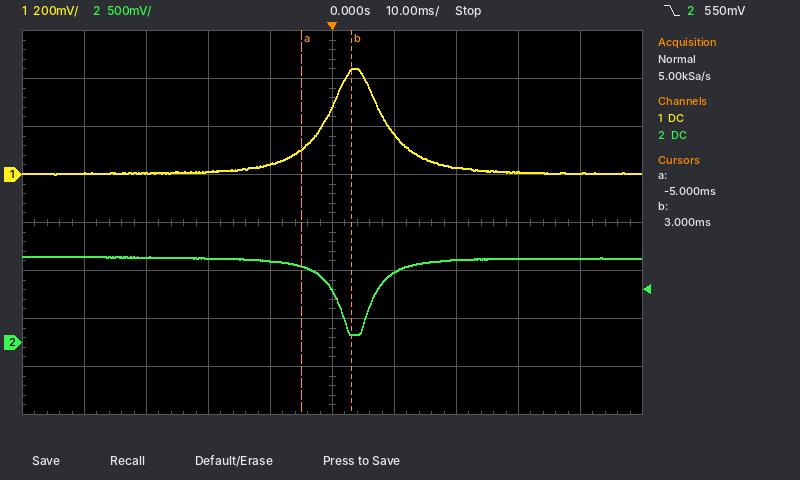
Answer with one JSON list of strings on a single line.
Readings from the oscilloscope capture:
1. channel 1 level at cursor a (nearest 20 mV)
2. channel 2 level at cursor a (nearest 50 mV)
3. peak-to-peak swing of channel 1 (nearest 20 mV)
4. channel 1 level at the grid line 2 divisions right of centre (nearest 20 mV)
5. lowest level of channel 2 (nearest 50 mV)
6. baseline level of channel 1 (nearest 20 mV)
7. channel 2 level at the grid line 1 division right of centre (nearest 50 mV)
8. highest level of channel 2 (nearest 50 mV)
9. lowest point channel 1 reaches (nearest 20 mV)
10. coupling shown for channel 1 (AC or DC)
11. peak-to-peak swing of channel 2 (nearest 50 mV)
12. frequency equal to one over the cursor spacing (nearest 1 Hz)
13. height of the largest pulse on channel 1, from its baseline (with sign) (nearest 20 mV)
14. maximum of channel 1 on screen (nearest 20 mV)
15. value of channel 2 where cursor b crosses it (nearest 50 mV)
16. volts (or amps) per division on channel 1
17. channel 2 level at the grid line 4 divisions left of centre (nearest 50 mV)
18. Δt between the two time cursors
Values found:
["100 mV", "800 mV", "440 mV", "20 mV", "100 mV", "0 mV", "750 mV", "900 mV", "0 mV", "DC", "800 mV", "125 Hz", "+440 mV", "440 mV", "100 mV", "200 mV", "900 mV", "8 ms"]
